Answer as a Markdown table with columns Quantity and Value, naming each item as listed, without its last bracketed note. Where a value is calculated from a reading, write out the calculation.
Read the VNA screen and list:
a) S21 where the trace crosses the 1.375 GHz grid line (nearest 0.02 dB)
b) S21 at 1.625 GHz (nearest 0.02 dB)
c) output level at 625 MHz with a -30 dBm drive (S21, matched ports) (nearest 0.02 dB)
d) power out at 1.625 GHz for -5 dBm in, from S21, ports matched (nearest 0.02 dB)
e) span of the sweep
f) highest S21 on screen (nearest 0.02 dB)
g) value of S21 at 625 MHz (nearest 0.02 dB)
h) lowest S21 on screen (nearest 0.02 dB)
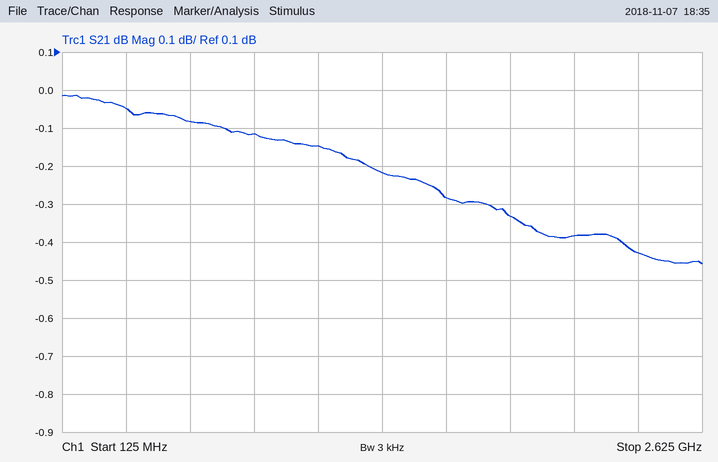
| Quantity | Value |
|---|---|
| S21 where the trace crosses the 1.375 GHz grid line | -0.22 dB |
| S21 at 1.625 GHz | -0.28 dB |
| output level at 625 MHz with a -30 dBm drive (S21, matched ports) | -30 dBm + (-0.08 dB) = -30.08 dBm |
| power out at 1.625 GHz for -5 dBm in, from S21, ports matched | -5 dBm + (-0.28 dB) = -5.28 dBm |
| span of the sweep | 2.5 GHz |
| highest S21 on screen | -0.02 dB |
| value of S21 at 625 MHz | -0.08 dB |
| lowest S21 on screen | -0.46 dB |
